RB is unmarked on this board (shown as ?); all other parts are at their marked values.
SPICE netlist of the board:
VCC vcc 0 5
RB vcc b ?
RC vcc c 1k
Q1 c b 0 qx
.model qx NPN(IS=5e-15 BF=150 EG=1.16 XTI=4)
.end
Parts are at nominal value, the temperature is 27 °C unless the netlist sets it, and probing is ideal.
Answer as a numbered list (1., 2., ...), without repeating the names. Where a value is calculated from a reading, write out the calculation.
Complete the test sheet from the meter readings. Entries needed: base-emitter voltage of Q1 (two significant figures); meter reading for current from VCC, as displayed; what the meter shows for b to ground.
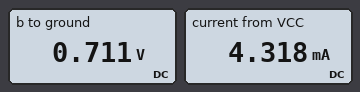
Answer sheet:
1. 711 mV = 710 mV
2. 4.318 mA
3. 0.711 V
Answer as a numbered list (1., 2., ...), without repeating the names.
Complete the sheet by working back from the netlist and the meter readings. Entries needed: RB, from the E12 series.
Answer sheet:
1. 150 kΩ
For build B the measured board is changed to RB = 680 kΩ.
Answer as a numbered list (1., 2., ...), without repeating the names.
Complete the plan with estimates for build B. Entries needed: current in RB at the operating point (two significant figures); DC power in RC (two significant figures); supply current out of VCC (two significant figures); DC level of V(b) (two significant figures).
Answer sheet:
1. 6.4 µA
2. 910 µW
3. 960 µA
4. 670 mV
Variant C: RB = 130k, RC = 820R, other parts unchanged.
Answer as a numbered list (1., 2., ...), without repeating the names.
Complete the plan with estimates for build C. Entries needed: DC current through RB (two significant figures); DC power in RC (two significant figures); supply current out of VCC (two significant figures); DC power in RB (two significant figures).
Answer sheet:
1. 33 µA
2. 20 mW
3. 5.0 mA
4. 140 µW
